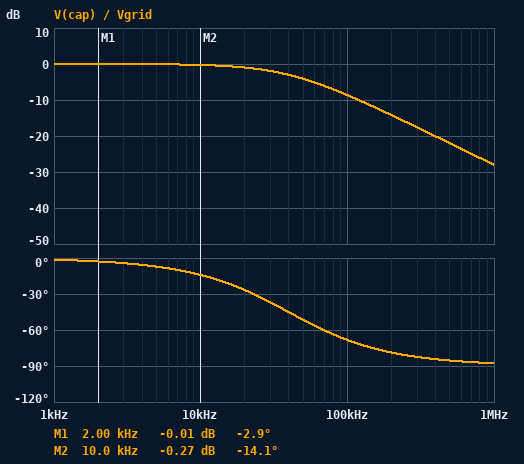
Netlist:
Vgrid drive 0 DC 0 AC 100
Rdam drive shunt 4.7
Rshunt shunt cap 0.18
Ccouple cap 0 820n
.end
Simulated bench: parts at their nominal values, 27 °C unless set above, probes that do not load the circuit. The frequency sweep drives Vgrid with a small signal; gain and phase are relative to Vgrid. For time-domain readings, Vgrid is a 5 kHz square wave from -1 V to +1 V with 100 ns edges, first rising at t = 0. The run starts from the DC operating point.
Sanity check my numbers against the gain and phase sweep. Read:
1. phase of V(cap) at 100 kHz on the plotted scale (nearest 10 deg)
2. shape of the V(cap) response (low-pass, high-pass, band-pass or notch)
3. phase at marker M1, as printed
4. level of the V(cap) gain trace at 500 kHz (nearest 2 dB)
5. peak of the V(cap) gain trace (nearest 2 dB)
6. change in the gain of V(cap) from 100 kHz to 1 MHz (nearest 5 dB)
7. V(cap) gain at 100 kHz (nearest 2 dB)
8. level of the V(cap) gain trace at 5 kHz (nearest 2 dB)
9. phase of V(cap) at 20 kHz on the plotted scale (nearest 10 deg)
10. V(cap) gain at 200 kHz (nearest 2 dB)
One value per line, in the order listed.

-70 deg
low-pass
-2.9 deg
-22 dB
0 dB
-20 dB
-8 dB
0 dB
-30 deg
-14 dB
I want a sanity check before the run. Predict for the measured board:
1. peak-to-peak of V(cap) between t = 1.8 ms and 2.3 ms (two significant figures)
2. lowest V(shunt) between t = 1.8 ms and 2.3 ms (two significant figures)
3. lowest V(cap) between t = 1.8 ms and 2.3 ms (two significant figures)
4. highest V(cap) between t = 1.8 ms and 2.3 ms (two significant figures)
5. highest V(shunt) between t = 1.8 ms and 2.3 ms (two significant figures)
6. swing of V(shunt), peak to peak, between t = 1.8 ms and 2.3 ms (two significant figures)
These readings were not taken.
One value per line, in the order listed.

2.0 V
-1.0 V
-1.0 V
1.0 V
1.0 V
2.0 V
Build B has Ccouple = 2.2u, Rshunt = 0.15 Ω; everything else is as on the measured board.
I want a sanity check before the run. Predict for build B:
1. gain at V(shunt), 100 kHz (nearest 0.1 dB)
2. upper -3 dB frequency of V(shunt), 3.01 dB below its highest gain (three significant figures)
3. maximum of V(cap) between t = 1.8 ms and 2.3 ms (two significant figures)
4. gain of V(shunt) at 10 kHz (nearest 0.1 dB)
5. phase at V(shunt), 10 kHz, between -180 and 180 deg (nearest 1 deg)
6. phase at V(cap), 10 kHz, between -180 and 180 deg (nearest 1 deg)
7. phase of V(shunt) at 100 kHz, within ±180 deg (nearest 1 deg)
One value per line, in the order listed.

-16.4 dB
14.9 kHz
1.0 V
-1.6 dB
-33 deg
-34 deg
-70 deg
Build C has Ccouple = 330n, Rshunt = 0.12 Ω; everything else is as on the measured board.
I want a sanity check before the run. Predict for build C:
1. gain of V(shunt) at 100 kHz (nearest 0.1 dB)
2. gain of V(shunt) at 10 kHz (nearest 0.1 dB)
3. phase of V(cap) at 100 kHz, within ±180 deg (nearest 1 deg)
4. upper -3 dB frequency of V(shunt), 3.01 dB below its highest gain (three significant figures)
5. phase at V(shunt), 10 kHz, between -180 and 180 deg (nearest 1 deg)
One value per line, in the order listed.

-3.0 dB
0 dB
-45 deg
100 kHz
-6 deg
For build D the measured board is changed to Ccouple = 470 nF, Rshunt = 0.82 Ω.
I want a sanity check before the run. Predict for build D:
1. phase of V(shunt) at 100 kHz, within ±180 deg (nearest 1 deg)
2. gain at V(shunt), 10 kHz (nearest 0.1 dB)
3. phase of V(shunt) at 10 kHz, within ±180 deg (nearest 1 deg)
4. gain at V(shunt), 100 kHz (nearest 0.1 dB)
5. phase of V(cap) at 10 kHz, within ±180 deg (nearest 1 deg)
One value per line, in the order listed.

-45 deg
-0.1 dB
-8 deg
-5.4 dB
-9 deg
